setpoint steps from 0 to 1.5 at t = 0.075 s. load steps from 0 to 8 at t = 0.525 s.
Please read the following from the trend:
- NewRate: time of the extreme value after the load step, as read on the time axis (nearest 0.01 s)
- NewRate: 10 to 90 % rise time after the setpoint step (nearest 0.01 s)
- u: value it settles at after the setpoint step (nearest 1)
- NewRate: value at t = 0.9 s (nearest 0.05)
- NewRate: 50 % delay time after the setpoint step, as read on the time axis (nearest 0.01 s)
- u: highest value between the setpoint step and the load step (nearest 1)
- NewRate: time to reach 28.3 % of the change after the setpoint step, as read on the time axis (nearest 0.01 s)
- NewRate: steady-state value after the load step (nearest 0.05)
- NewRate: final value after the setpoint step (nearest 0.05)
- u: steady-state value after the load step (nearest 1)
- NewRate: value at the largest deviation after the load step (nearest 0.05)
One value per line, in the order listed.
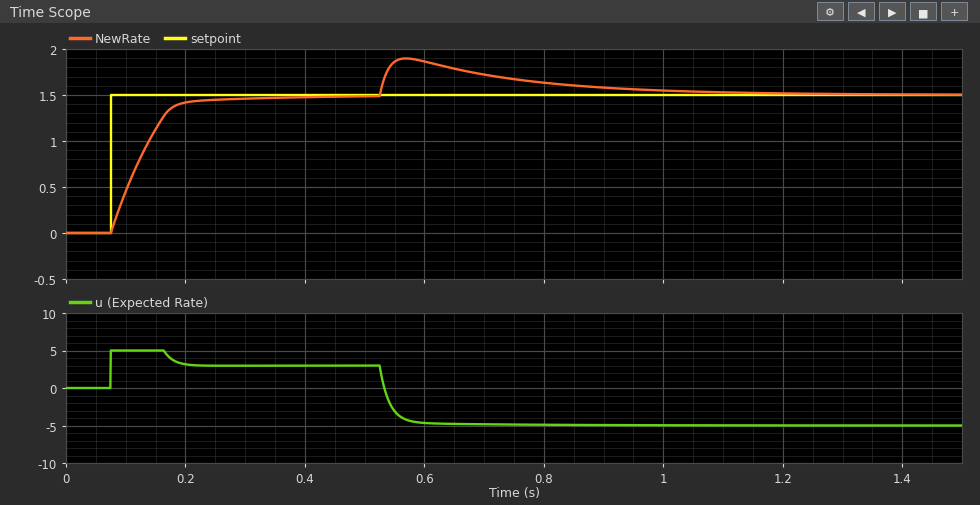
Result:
0.57 s
0.09 s
3
1.60
0.12 s
5
0.10 s
1.50
1.50
-5
1.90
